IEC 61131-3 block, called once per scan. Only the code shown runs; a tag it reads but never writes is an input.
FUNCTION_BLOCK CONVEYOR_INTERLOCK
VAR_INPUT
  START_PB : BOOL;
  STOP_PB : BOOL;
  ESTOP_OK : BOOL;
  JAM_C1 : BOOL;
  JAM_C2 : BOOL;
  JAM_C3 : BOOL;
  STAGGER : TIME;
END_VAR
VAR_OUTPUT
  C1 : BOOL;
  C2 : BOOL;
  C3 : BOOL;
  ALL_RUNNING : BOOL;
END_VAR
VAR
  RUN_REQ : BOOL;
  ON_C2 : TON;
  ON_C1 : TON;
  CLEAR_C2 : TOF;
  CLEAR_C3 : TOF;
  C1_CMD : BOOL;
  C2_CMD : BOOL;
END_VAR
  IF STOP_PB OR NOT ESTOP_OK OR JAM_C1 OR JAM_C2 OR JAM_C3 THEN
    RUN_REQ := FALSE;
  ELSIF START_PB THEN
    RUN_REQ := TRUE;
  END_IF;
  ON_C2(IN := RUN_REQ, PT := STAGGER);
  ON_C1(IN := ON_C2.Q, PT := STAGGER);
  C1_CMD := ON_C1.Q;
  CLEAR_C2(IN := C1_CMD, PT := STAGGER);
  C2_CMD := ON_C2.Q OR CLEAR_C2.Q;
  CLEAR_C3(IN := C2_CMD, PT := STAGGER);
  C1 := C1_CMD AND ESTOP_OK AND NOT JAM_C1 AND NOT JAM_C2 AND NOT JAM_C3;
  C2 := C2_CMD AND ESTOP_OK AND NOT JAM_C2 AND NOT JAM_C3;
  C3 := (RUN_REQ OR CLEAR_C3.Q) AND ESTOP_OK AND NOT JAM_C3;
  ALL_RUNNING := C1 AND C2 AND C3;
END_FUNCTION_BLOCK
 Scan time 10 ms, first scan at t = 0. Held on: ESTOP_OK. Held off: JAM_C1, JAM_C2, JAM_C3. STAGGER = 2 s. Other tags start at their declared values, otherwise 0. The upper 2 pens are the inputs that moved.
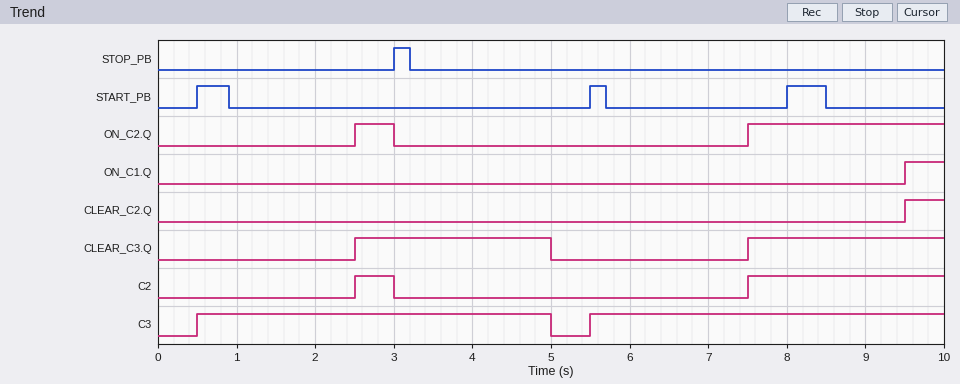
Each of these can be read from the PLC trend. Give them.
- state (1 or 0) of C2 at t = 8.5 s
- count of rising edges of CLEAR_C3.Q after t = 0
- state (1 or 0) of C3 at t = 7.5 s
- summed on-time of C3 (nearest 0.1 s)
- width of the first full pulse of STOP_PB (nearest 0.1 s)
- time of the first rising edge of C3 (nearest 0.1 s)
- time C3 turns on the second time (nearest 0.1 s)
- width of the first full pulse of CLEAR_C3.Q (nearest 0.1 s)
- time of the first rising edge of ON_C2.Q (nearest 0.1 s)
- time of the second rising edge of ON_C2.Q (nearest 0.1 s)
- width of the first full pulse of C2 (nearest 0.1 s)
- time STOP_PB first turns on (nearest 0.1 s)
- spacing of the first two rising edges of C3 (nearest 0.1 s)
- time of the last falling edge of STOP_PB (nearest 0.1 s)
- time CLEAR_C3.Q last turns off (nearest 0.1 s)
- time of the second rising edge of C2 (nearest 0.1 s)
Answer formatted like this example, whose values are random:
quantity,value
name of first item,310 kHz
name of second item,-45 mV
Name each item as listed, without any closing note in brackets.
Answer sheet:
quantity,value
state (1 or 0) of C2 at t = 8.5 s,1
count of rising edges of CLEAR_C3.Q after t = 0,2
state (1 or 0) of C3 at t = 7.5 s,1
summed on-time of C3,9.0 s
width of the first full pulse of STOP_PB,0.2 s
time of the first rising edge of C3,0.5 s
time C3 turns on the second time,5.5 s
width of the first full pulse of CLEAR_C3.Q,2.5 s
time of the first rising edge of ON_C2.Q,2.5 s
time of the second rising edge of ON_C2.Q,7.5 s
width of the first full pulse of C2,0.5 s
time STOP_PB first turns on,3.0 s
spacing of the first two rising edges of C3,5.0 s
time of the last falling edge of STOP_PB,3.2 s
time CLEAR_C3.Q last turns off,5.0 s
time of the second rising edge of C2,7.5 s
